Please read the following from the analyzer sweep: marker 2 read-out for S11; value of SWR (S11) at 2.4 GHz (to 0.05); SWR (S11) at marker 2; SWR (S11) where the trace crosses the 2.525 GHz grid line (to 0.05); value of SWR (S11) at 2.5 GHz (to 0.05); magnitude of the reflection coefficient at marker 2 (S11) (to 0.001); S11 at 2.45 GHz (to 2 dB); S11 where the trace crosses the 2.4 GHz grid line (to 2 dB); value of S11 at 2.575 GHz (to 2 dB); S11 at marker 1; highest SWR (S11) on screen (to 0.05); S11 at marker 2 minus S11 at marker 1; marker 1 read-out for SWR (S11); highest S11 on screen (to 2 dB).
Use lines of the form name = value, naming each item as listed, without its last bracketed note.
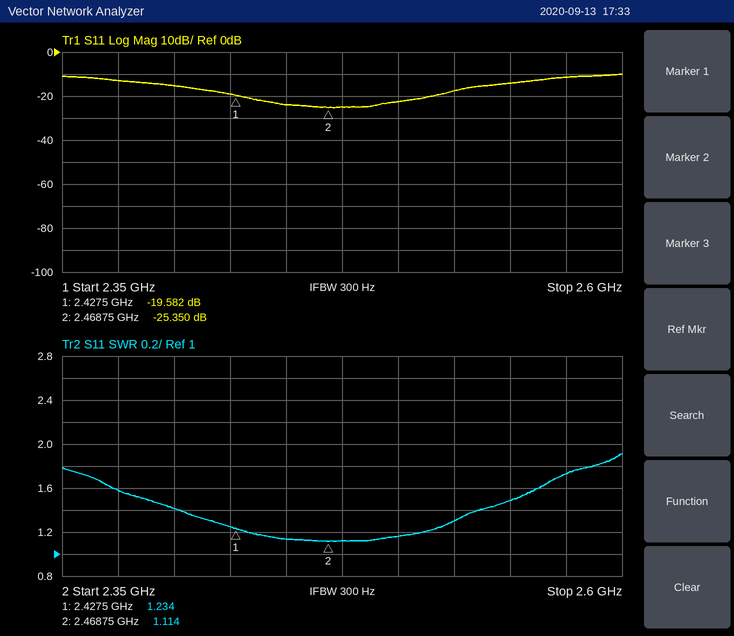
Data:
marker 2 read-out for S11 = -25.350 dB
value of SWR (S11) at 2.4 GHz = 1.40
SWR (S11) at marker 2 = 1.114
SWR (S11) where the trace crosses the 2.525 GHz grid line = 1.30
value of SWR (S11) at 2.5 GHz = 1.15
magnitude of the reflection coefficient at marker 2 (S11) = 0.054
S11 at 2.45 GHz = -24 dB
S11 where the trace crosses the 2.4 GHz grid line = -16 dB
value of S11 at 2.575 GHz = -12 dB
S11 at marker 1 = -19.582 dB
highest SWR (S11) on screen = 1.90
S11 at marker 2 minus S11 at marker 1 = -5.768 dB
marker 1 read-out for SWR = 1.234
highest S11 on screen = -10 dB
